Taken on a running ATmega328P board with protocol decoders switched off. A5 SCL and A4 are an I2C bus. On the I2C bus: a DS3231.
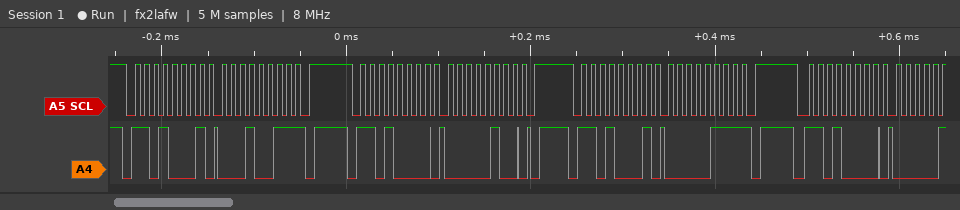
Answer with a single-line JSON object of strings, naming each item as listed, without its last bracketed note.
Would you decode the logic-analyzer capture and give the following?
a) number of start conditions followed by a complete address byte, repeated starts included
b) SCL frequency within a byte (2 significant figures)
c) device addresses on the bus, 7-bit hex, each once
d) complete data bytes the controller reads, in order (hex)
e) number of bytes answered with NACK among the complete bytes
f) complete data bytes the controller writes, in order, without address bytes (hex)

{"number of start conditions followed by a complete address byte, repeated starts included": "4", "SCL frequency within a byte": "100 kHz", "device addresses on the bus, 7-bit hex, each once": "0x68", "complete data bytes the controller reads, in order": "13 07", "number of bytes answered with NACK among the complete bytes": "2", "complete data bytes the controller writes, in order, without address bytes": "04"}
